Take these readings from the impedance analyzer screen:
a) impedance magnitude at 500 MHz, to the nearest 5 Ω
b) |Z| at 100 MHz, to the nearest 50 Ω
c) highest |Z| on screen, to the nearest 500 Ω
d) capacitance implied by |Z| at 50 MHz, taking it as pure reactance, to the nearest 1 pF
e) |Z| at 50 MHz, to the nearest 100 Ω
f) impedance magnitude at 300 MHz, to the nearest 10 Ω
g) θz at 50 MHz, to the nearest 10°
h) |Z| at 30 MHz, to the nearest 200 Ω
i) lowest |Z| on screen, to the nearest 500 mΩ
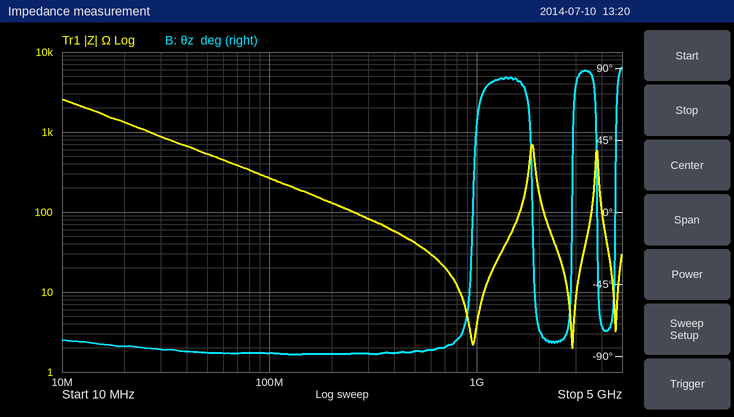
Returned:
40 Ω
250 Ω
2.5 kΩ
6 pF
500 Ω
80 Ω
-90°
800 Ω
2.0 Ω
